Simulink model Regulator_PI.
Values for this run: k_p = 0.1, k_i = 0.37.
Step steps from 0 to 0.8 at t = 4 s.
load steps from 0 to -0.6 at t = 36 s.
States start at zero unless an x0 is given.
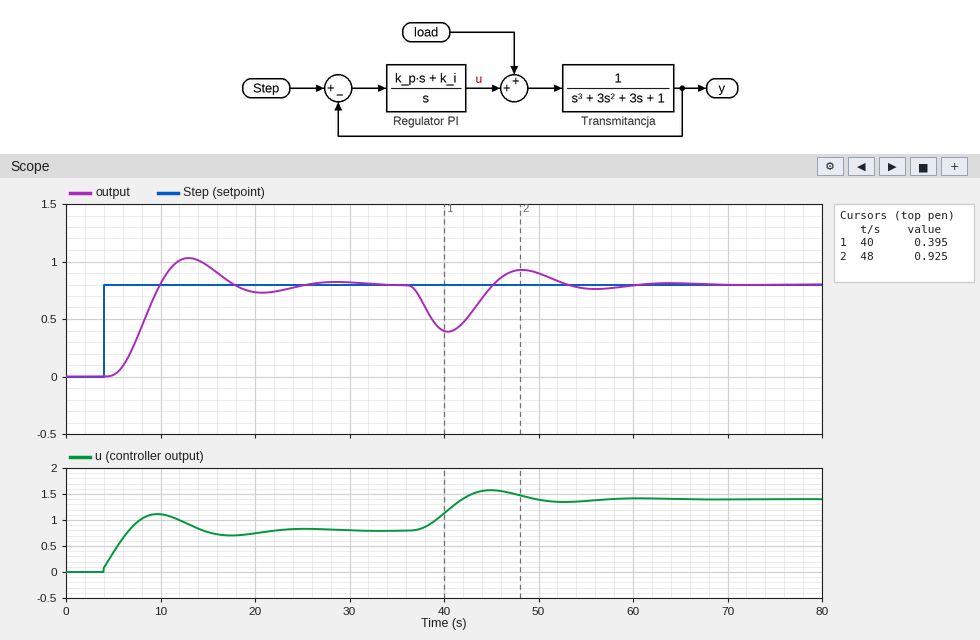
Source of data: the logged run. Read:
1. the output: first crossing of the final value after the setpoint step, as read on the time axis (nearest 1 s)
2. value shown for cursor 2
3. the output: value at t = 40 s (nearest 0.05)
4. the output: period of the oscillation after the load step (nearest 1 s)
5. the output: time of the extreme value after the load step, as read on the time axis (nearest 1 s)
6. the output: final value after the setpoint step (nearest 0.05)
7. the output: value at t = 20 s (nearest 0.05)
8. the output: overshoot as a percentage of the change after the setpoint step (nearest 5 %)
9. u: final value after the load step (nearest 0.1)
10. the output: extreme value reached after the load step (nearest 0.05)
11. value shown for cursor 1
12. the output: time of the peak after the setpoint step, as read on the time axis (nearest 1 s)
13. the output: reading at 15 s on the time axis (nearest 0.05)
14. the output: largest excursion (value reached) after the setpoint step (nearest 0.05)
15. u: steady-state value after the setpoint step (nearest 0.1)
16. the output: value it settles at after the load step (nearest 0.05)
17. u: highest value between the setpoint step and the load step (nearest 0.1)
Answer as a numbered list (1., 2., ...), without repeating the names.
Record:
1. 10 s
2. 0.925
3. 0.40
4. 16 s
5. 40 s
6. 0.80
7. 0.75
8. 30 %
9. 1.4
10. 0.40
11. 0.395
12. 13 s
13. 0.95
14. 1.05
15. 0.8
16. 0.80
17. 1.1
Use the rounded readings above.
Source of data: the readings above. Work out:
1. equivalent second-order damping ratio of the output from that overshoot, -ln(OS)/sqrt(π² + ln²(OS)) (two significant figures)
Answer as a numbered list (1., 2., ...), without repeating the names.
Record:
1. 0.36
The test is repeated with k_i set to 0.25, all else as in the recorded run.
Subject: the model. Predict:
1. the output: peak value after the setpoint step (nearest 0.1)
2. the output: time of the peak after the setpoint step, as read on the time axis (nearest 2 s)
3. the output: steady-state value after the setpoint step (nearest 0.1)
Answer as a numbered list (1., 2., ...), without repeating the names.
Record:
1. 0.9
2. 16 s
3. 0.8
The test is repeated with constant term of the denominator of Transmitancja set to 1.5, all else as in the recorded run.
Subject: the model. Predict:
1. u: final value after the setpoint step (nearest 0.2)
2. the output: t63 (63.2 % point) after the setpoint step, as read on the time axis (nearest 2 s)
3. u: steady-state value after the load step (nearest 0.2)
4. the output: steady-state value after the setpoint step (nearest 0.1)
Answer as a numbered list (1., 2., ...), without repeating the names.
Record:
1. 1.2
2. 8 s
3. 1.8
4. 0.8
